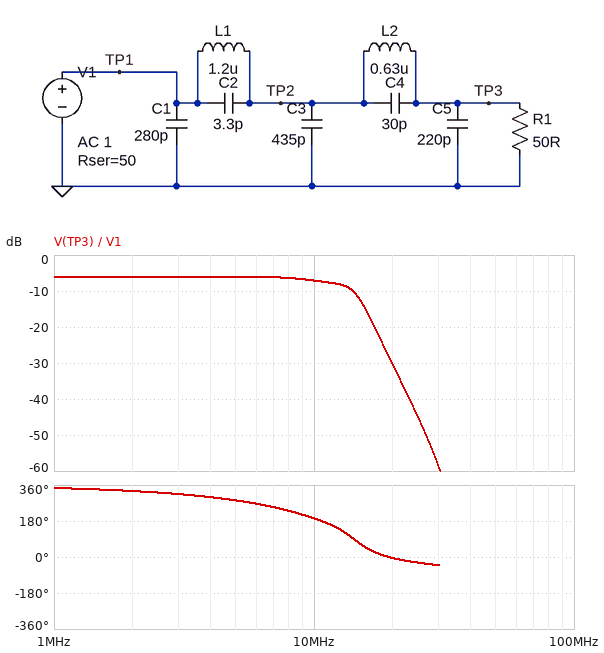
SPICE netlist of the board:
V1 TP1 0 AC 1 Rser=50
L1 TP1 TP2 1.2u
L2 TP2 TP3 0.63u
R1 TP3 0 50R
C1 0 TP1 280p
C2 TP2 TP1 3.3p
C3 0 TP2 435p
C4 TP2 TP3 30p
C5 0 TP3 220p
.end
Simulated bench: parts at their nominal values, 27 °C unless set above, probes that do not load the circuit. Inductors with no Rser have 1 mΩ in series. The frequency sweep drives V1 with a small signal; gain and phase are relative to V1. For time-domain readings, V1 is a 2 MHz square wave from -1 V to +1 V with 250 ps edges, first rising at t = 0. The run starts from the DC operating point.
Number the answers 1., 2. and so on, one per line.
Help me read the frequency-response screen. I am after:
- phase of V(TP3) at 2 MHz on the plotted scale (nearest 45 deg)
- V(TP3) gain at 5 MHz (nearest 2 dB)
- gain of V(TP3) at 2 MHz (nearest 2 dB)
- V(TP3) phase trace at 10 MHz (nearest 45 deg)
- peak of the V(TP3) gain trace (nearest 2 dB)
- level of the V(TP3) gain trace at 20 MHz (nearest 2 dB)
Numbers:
1. 315 deg
2. -6 dB
3. -6 dB
4. 180 deg
5. -6 dB
6. -30 dB
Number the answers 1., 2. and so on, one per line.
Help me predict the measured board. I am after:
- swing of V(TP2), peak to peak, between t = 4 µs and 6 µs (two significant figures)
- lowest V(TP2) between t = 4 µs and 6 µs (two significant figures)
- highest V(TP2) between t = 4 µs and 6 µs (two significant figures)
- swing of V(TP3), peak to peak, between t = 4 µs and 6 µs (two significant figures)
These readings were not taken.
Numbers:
1. 1.1 V
2. -570 mV
3. 570 mV
4. 1.3 V
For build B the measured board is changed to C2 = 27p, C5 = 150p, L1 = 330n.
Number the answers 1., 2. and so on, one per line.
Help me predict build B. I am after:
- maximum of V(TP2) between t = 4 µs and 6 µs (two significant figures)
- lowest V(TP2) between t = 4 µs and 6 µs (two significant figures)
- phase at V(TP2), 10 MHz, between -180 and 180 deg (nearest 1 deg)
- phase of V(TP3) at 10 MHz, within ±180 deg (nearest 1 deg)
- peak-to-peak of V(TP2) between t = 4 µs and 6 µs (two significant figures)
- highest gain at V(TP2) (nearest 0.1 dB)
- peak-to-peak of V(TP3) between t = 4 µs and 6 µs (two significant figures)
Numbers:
1. 650 mV
2. -650 mV
3. -56 deg
4. -111 deg
5. 1.3 V
6. -1.9 dB
7. 1.2 V
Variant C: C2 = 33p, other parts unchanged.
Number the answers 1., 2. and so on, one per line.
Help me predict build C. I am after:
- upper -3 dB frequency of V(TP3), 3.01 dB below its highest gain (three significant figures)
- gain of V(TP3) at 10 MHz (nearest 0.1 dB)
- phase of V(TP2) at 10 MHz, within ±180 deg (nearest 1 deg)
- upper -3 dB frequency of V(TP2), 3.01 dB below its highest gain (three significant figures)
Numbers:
1. 11.3 MHz
2. -7.9 dB
3. -111 deg
4. 11.6 MHz
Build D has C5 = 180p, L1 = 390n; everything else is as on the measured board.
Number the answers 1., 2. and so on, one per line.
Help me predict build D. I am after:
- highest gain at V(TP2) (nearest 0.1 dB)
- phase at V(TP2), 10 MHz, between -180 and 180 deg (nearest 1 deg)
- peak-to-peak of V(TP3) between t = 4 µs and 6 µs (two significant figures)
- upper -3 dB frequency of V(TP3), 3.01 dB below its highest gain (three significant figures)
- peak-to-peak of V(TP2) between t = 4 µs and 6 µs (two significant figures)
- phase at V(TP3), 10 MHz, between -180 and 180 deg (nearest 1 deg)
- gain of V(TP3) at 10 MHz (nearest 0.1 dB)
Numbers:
1. -1.6 dB
2. -57 deg
3. 1.2 V
4. 18.9 MHz
5. 1.3 V
6. -116 deg
7. -6.7 dB
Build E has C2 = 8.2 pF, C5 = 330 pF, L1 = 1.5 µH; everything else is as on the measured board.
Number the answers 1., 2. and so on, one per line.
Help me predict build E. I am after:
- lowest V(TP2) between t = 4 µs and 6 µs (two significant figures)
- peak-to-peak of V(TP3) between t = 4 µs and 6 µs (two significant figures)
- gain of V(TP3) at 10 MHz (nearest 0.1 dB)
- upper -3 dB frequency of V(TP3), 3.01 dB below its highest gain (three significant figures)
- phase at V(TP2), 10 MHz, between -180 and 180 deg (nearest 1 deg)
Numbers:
1. -560 mV
2. 1.2 V
3. -9.2 dB
4. 9.68 MHz
5. -103 deg
